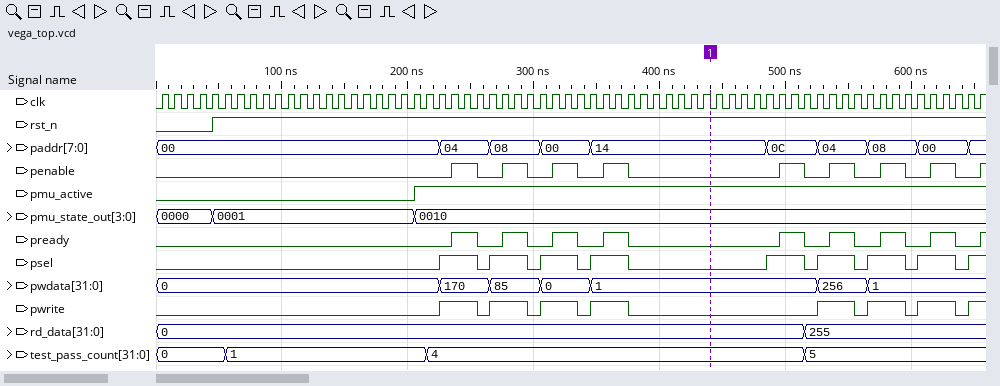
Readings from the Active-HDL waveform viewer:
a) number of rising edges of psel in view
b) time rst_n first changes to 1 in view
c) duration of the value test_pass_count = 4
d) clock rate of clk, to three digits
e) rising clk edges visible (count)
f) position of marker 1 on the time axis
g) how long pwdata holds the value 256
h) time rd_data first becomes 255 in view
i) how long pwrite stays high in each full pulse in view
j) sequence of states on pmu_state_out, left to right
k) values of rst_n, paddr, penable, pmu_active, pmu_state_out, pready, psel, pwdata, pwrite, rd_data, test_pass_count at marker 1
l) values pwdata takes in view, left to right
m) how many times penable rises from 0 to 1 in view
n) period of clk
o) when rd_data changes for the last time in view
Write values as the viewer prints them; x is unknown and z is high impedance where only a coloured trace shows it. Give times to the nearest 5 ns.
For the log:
9
45 ns
300 ns
100 MHz
66
440 ns
40 ns
515 ns
30 ns, 30 ns, 30 ns, 30 ns, 30 ns, 30 ns, 30 ns
0000, 0001, 0010
rst_n=1, paddr=14, penable=0, pmu_active=1, pmu_state_out=0010, pready=0, psel=0, pwdata=1, pwrite=0, rd_data=0, test_pass_count=4
0, 170, 85, 0, 1, 256, 1
9
10 ns
515 ns
